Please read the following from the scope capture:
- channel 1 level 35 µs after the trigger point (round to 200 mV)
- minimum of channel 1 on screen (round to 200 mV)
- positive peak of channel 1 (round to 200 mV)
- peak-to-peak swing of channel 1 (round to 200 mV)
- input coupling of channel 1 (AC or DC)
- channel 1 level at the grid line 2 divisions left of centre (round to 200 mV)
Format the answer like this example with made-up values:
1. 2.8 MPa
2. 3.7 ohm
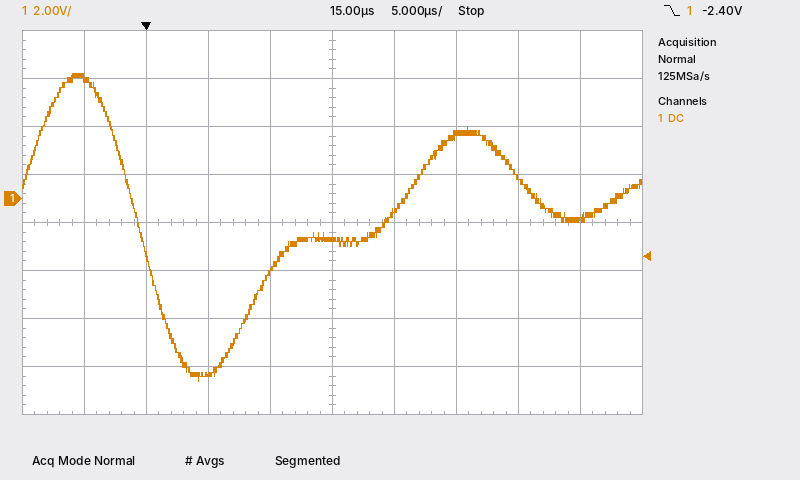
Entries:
1. -800 mV
2. -7.6 V
3. 5.2 V
4. 12.8 V
5. DC
6. -7.4 V
